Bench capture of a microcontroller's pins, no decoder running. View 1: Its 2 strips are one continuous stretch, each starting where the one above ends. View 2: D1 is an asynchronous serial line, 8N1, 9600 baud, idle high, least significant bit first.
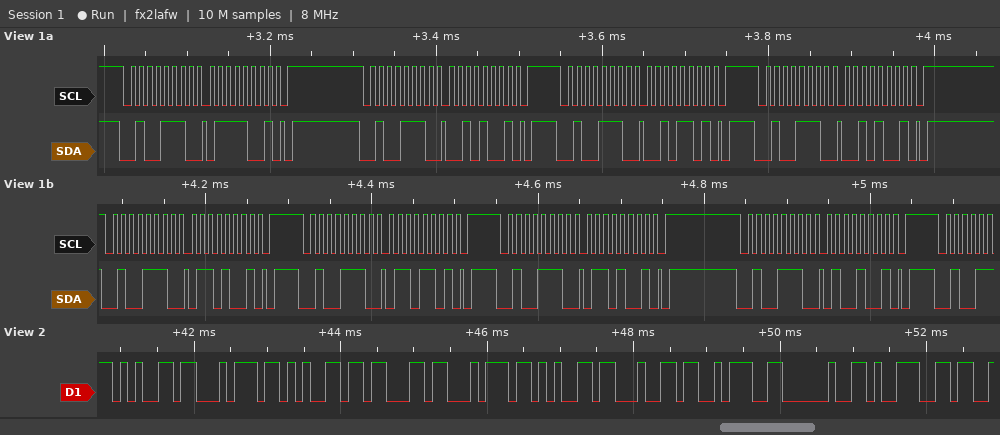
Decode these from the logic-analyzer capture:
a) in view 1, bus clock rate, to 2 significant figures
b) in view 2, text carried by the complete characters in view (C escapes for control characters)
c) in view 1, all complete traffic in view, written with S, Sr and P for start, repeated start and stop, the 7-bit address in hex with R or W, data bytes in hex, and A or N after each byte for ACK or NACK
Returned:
100 kHz
"etected: 9"
S 27W A 79 A P S 27W A 29 A P S 27W A 2D A P S 27W A 29 A P S 27W A 69 A P S 27W A 6D A P S 27W A 69 A P S 27W A 49 A P
